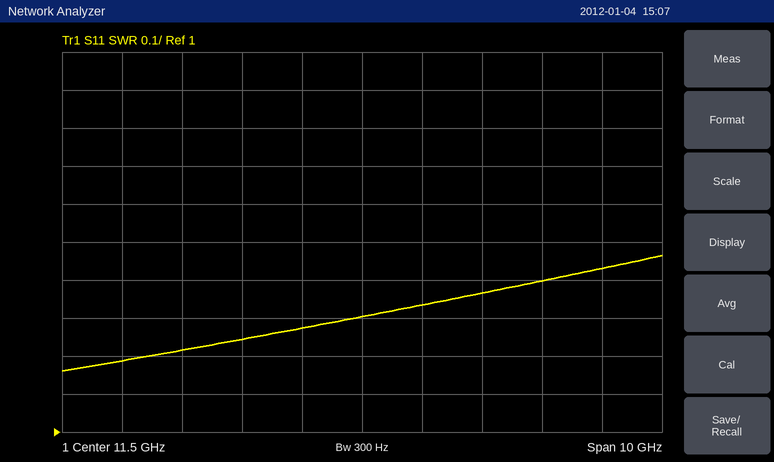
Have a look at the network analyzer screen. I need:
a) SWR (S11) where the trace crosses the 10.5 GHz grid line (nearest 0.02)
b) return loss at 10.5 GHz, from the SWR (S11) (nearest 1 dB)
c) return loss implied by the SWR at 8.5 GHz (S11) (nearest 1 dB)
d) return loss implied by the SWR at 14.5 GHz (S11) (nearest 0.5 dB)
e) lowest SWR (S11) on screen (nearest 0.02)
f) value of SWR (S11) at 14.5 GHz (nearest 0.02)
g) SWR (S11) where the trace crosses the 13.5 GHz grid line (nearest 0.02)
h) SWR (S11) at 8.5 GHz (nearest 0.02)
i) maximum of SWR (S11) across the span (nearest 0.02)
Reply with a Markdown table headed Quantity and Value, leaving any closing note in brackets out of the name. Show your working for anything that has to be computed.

| Quantity | Value |
|---|---|
| SWR (S11) where the trace crosses the 10.5 GHz grid line | 1.28 |
| return loss at 10.5 GHz, from the SWR (S11) | −20 log10((1.28 − 1)/(1.28 + 1)) ≈ 18 dB |
| return loss implied by the SWR at 8.5 GHz (S11) | −20 log10((1.22 − 1)/(1.22 + 1)) ≈ 20 dB |
| return loss implied by the SWR at 14.5 GHz (S11) | −20 log10((1.4 − 1)/(1.4 + 1)) ≈ 15.6 dB, so 15.5 dB to the nearest 0.5 dB |
| lowest SWR (S11) on screen | 1.16 |
| value of SWR (S11) at 14.5 GHz | 1.40 |
| SWR (S11) where the trace crosses the 13.5 GHz grid line | 1.36 |
| SWR (S11) at 8.5 GHz | 1.22 |
| maximum of SWR (S11) across the span | 1.46 |
